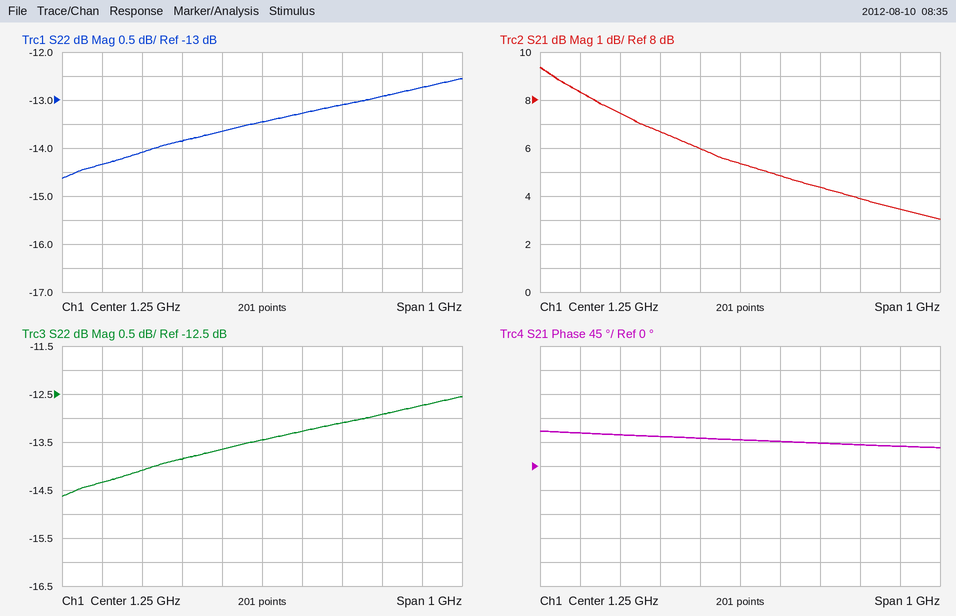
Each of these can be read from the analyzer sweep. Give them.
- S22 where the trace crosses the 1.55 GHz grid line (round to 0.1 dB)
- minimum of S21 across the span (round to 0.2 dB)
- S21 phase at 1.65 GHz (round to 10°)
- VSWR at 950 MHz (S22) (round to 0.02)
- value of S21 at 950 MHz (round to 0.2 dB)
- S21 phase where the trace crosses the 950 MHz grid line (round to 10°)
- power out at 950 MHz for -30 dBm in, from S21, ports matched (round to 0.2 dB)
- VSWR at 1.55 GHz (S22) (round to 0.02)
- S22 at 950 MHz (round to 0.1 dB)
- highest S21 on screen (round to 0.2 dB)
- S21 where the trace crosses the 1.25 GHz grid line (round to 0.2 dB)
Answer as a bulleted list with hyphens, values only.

- -12.9 dB
- 3.0 dB
- 40°
- 1.50
- 7.4 dB
- 60°
- -22.6 dBm
- 1.58
- -14.1 dB
- 9.4 dB
- 5.4 dB
